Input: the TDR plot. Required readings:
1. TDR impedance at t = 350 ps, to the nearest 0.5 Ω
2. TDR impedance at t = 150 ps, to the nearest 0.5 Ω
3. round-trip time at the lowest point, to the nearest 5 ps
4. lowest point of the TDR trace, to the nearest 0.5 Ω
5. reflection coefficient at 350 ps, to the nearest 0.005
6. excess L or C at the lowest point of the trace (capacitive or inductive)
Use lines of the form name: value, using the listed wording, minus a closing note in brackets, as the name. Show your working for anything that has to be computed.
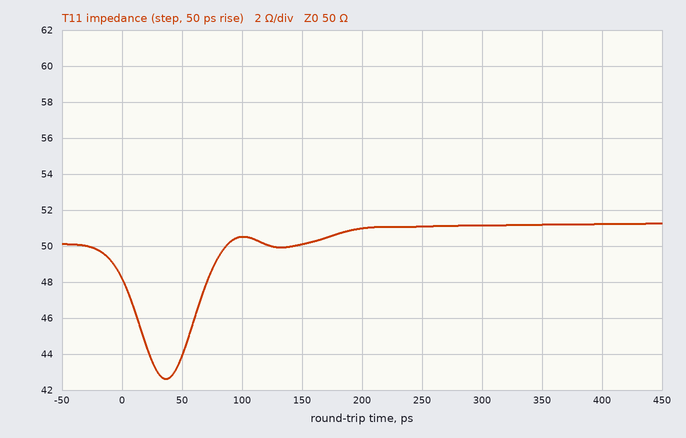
TDR impedance at t = 350 ps, to the nearest 0.5 Ω: 51.0 Ω
TDR impedance at t = 150 ps, to the nearest 0.5 Ω: 50.0 Ω
round-trip time at the lowest point, to the nearest 5 ps: 35 ps
lowest point of the TDR trace, to the nearest 0.5 Ω: 42.5 Ω
reflection coefficient at 350 ps, to the nearest 0.005: (51 − 50)/(51 + 50) ≈ +0.010
excess L or C at the lowest point of the trace: capacitive
